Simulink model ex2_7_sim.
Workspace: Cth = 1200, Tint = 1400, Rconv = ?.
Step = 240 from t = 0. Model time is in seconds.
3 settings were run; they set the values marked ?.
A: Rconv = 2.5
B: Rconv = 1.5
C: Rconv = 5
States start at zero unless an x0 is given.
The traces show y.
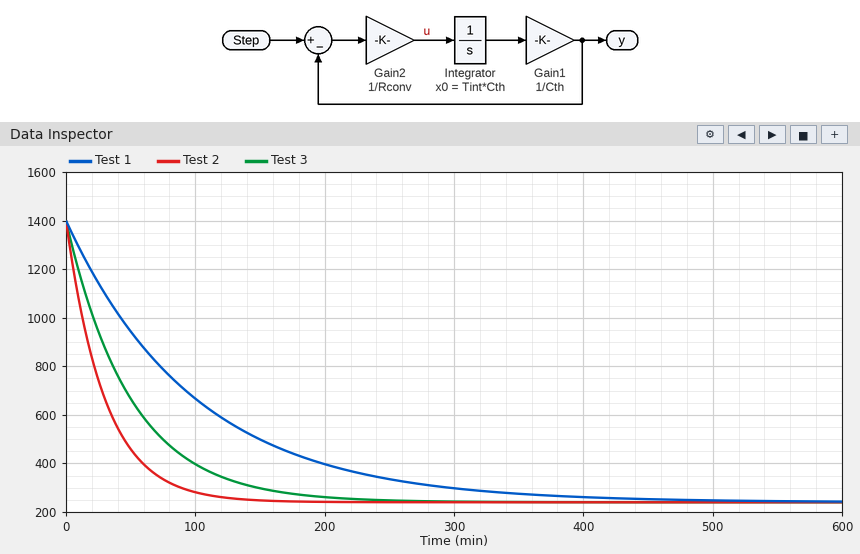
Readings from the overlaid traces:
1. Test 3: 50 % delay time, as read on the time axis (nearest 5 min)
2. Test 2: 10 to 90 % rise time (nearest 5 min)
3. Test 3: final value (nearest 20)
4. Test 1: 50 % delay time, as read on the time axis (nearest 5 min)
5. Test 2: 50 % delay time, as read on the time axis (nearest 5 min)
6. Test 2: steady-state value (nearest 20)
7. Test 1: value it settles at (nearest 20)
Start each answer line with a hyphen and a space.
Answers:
- 35 min
- 65 min
- 240
- 70 min
- 20 min
- 240
- 240
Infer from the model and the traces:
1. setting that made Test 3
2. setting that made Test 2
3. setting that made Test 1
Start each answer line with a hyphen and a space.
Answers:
- A
- B
- C
